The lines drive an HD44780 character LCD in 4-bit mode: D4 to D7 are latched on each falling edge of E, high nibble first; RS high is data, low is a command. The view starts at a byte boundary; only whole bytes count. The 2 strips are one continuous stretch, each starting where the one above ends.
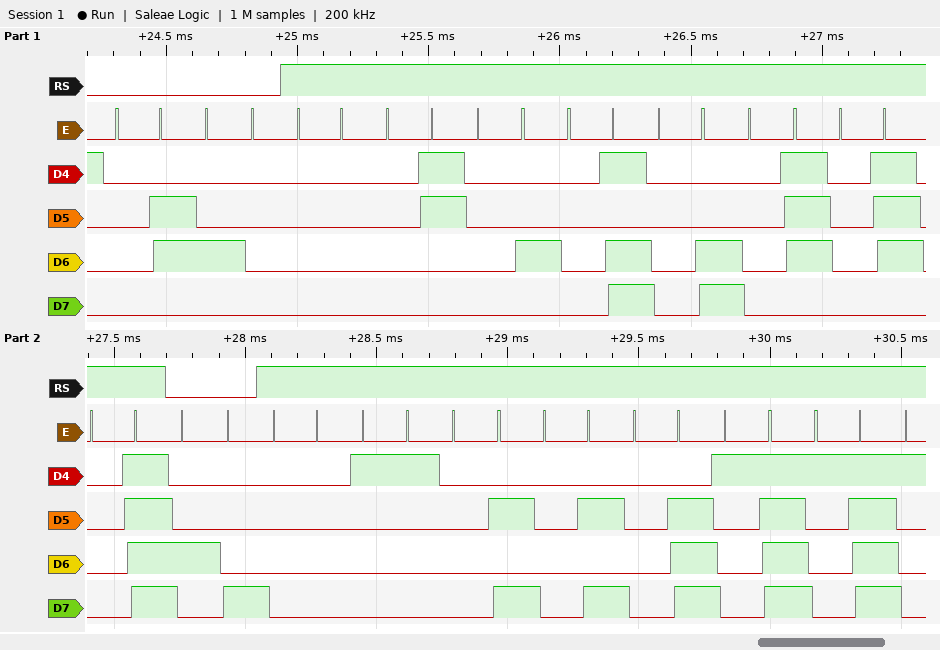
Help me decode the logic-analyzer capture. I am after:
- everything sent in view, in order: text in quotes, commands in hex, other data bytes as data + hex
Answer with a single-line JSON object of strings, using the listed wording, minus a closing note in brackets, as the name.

{"everything sent in view, in order: text in quotes, commands in hex, other data bytes as data + hex": "0x06 0x40 data 00 03 04 0D 0C 07 07 0F 0x48 data 00 11 0A 0A 0E 1F 1F"}
